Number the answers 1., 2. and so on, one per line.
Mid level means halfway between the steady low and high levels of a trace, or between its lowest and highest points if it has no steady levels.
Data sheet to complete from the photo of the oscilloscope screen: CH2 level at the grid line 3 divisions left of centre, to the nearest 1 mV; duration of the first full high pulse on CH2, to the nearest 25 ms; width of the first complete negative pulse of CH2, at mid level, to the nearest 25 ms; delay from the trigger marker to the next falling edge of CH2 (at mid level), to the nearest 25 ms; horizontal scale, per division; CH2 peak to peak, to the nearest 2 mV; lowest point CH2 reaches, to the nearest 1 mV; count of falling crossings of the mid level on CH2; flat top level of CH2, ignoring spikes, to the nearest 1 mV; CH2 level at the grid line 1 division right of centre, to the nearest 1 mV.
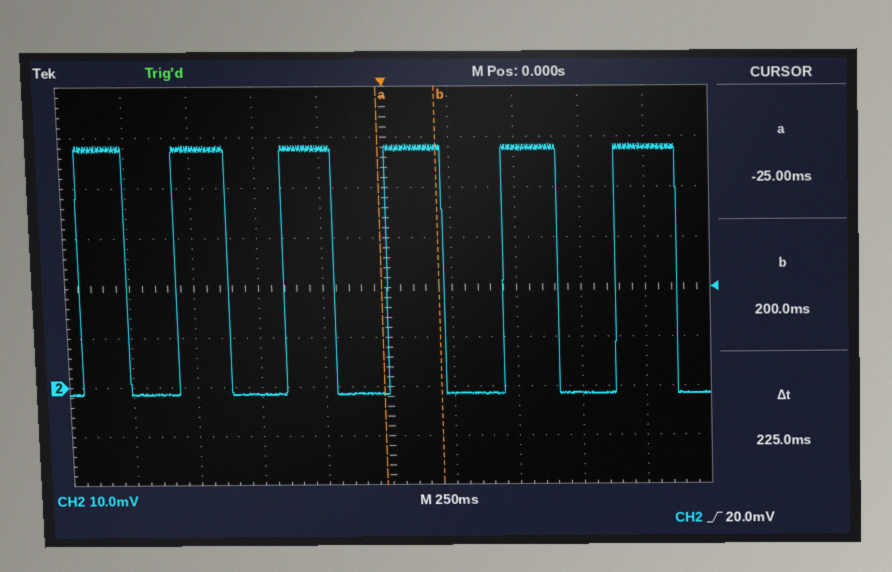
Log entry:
1. 48 mV
2. 175 ms
3. 200 ms
4. 225 ms
5. 250 ms
6. 50 mV
7. -2 mV
8. 6
9. 48 mV
10. -1 mV
